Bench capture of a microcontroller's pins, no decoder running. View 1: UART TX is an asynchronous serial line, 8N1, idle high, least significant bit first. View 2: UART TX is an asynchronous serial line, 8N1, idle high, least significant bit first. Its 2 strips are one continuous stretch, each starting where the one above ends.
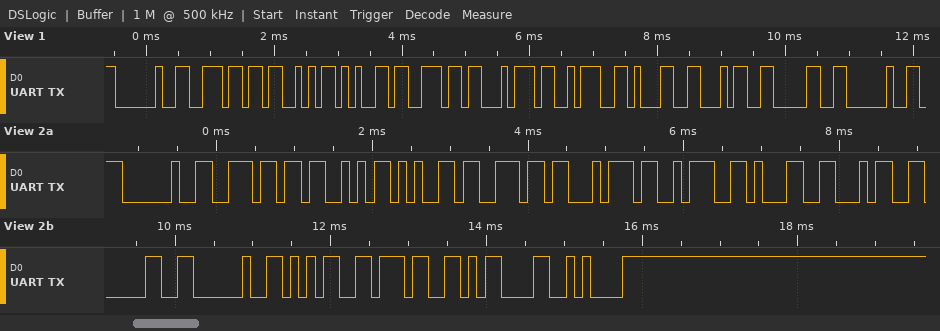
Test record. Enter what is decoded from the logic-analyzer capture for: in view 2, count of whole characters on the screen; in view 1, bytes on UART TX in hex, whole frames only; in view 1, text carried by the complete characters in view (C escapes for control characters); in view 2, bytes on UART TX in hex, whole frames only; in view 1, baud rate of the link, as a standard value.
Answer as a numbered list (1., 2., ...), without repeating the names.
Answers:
1. 15
2. 20 6E 53 65 6E 74 3A 31 34 30 20
3. " nSent:140 "
4. 20 6E 53 65 6E 74 3A 31 34 30 20 35 37 0D 0A
5. 9600 baud
